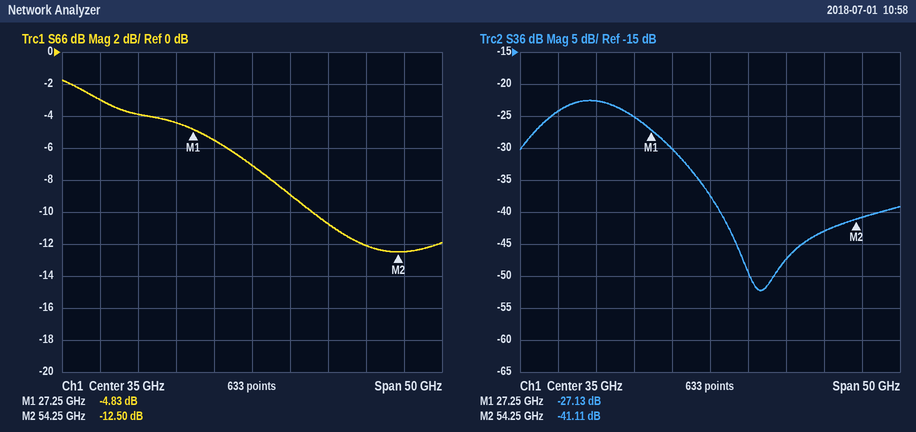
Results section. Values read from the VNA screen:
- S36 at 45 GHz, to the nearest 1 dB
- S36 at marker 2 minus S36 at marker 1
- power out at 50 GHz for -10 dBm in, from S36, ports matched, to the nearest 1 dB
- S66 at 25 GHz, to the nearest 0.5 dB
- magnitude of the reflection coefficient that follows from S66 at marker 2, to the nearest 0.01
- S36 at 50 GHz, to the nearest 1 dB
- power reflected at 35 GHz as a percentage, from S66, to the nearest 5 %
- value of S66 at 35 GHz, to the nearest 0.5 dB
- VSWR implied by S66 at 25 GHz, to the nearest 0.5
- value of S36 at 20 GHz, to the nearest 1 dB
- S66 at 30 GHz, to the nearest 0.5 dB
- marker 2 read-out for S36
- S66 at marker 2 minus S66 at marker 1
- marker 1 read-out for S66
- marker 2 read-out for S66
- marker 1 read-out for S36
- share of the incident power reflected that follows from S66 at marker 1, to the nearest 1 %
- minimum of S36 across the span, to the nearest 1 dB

-47 dB
-13.98 dB
-53 dBm
-4.5 dB
0.24
-43 dB
20 %
-7.0 dB
4.0
-23 dB
-5.5 dB
-41.11 dB
-7.67 dB
-4.83 dB
-12.50 dB
-27.13 dB
33 %
-52 dB
